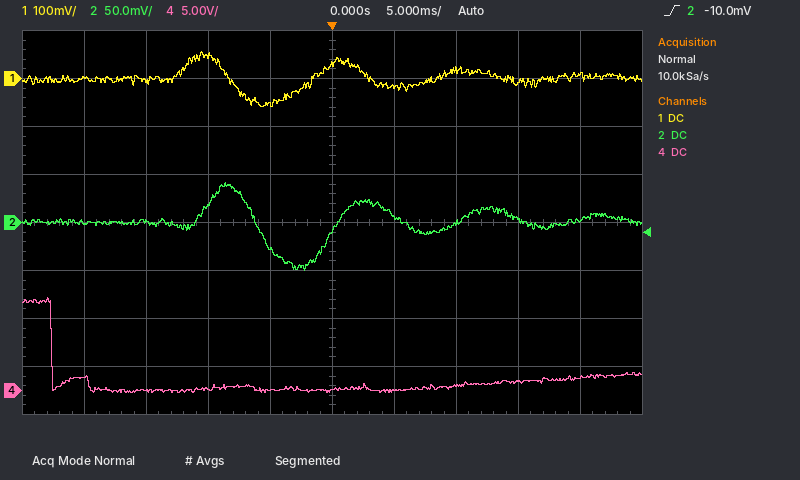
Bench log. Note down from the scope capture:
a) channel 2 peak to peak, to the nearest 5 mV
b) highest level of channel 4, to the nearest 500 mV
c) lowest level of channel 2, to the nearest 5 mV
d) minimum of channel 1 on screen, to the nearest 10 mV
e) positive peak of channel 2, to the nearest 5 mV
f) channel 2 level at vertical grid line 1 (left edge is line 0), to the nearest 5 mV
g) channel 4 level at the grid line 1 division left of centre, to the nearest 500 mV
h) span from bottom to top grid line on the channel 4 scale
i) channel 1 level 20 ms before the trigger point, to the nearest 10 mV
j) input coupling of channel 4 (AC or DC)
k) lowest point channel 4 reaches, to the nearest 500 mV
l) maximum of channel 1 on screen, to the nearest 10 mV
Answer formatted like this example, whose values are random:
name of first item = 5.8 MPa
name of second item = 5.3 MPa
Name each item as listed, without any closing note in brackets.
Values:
channel 2 peak to peak, to the nearest 5 mV = 90 mV
highest level of channel 4, to the nearest 500 mV = 9.5 V
lowest level of channel 2, to the nearest 5 mV = -50 mV
minimum of channel 1 on screen, to the nearest 10 mV = -60 mV
positive peak of channel 2, to the nearest 5 mV = 40 mV
channel 2 level at vertical grid line 1 (left edge is line 0), to the nearest 5 mV = 0 mV
channel 4 level at the grid line 1 division left of centre, to the nearest 500 mV = 0.0 V
span from bottom to top grid line on the channel 4 scale = 40 V
channel 1 level 20 ms before the trigger point, to the nearest 10 mV = 0 mV
input coupling of channel 4 = DC
lowest point channel 4 reaches, to the nearest 500 mV = 0.0 V
maximum of channel 1 on screen, to the nearest 10 mV = 60 mV
